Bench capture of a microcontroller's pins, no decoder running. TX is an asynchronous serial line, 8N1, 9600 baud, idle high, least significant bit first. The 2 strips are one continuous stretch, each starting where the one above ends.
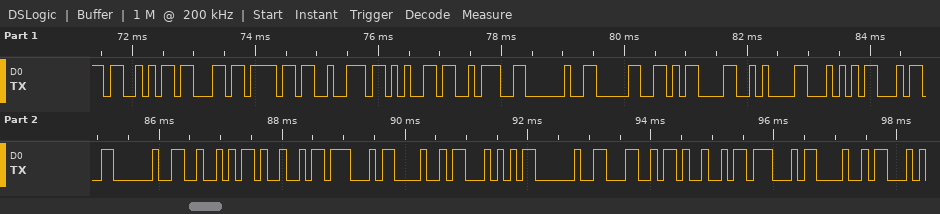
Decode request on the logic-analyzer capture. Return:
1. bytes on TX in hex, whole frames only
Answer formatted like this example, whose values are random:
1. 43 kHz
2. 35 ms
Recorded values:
1. 0x53 0x63 0x6F 0x72 0x65 0x3A 0x20 0x30 0x0D 0x0A 0x54 0x34 0x20 0x52 0x49 0x47 0x48 0x54 0x20 0x4C 0x49 0x47 0x48
